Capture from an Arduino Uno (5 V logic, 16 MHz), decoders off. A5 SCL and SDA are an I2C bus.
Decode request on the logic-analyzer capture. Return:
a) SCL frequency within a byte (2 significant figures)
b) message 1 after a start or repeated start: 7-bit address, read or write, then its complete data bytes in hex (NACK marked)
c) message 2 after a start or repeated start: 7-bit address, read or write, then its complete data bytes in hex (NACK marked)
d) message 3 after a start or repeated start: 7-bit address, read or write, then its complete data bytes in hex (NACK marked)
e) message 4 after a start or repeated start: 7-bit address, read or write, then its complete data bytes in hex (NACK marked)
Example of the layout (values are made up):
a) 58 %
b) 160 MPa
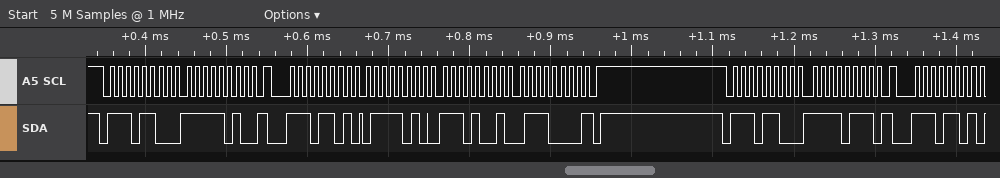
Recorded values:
a) 100 kHz
b) 0x76 write: FA
c) 0x76 read: 7A E9 70 NACK
d) 0x76 write: F7
e) 0x76 read
